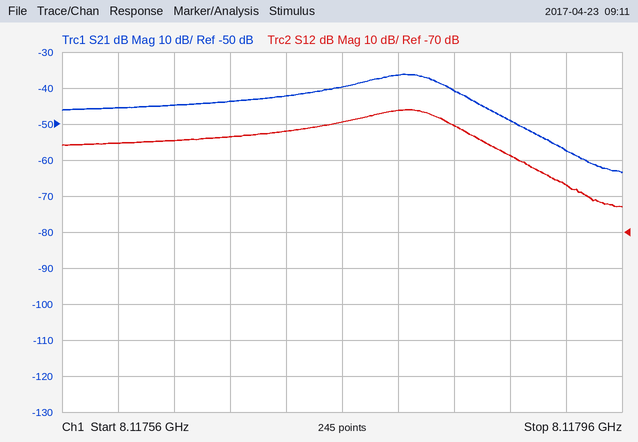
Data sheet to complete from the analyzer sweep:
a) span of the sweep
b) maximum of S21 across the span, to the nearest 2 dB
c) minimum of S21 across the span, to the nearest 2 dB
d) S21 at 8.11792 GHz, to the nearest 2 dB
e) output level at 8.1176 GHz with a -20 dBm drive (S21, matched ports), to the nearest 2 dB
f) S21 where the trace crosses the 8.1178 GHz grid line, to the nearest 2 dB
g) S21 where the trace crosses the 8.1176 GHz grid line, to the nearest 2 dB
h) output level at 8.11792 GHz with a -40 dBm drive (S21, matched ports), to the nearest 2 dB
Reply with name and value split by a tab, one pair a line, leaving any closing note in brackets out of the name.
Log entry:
span of the sweep	400 kHz
maximum of S21 across the span, to the nearest 2 dB	-36 dB
minimum of S21 across the span, to the nearest 2 dB	-64 dB
S21 at 8.11792 GHz, to the nearest 2 dB	-58 dB
output level at 8.1176 GHz with a -20 dBm drive (S21, matched ports), to the nearest 2 dB	-66 dBm
S21 where the trace crosses the 8.1178 GHz grid line, to the nearest 2 dB	-36 dB
S21 where the trace crosses the 8.1176 GHz grid line, to the nearest 2 dB	-46 dB
output level at 8.11792 GHz with a -40 dBm drive (S21, matched ports), to the nearest 2 dB	-98 dBm
